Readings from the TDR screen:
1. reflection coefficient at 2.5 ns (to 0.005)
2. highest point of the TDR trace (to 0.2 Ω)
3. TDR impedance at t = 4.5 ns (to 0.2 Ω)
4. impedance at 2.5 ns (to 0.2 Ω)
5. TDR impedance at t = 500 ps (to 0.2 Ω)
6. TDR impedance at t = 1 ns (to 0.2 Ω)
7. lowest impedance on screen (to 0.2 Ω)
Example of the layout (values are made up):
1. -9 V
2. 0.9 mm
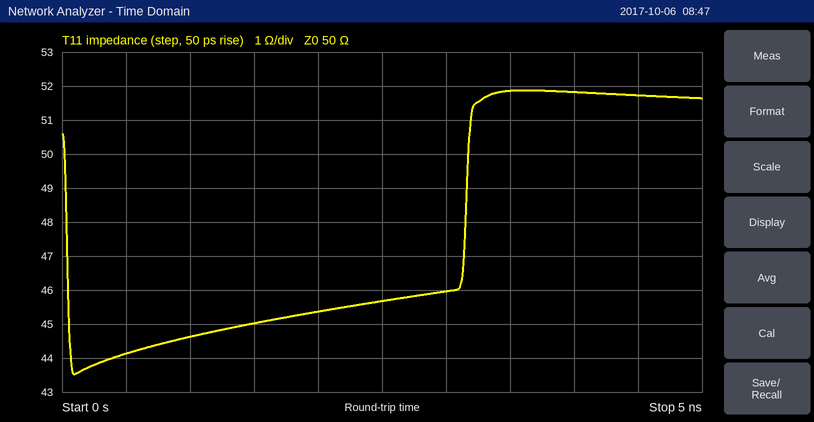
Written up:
1. -0.045
2. 51.8 Ω
3. 51.8 Ω
4. 45.6 Ω
5. 44.2 Ω
6. 44.6 Ω
7. 43.6 Ω
